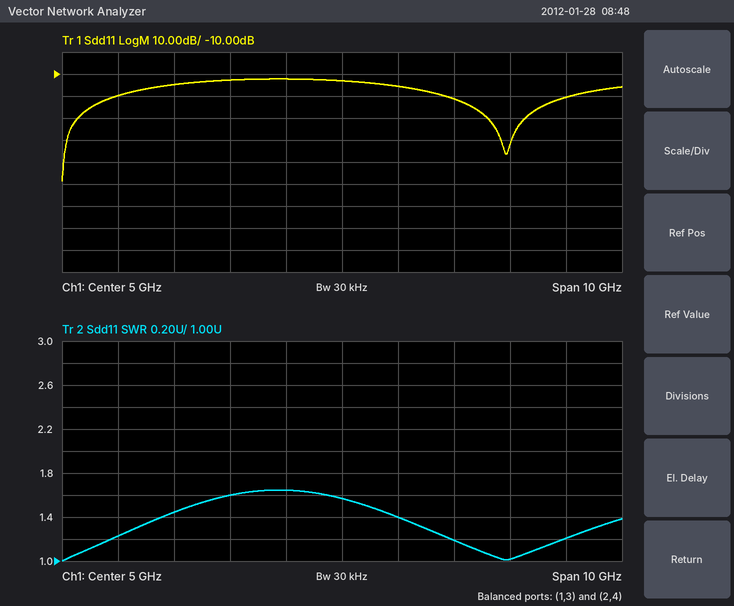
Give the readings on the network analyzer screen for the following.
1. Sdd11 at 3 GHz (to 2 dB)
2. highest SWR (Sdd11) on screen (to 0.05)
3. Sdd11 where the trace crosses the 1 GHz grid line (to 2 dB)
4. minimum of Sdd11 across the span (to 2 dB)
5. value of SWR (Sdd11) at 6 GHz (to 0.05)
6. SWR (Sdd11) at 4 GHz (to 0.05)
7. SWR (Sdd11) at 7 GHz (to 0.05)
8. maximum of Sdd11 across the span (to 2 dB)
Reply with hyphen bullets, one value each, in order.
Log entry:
- -12 dB
- 1.65
- -20 dB
- -58 dB
- 1.40
- 1.65
- 1.20
- -12 dB
